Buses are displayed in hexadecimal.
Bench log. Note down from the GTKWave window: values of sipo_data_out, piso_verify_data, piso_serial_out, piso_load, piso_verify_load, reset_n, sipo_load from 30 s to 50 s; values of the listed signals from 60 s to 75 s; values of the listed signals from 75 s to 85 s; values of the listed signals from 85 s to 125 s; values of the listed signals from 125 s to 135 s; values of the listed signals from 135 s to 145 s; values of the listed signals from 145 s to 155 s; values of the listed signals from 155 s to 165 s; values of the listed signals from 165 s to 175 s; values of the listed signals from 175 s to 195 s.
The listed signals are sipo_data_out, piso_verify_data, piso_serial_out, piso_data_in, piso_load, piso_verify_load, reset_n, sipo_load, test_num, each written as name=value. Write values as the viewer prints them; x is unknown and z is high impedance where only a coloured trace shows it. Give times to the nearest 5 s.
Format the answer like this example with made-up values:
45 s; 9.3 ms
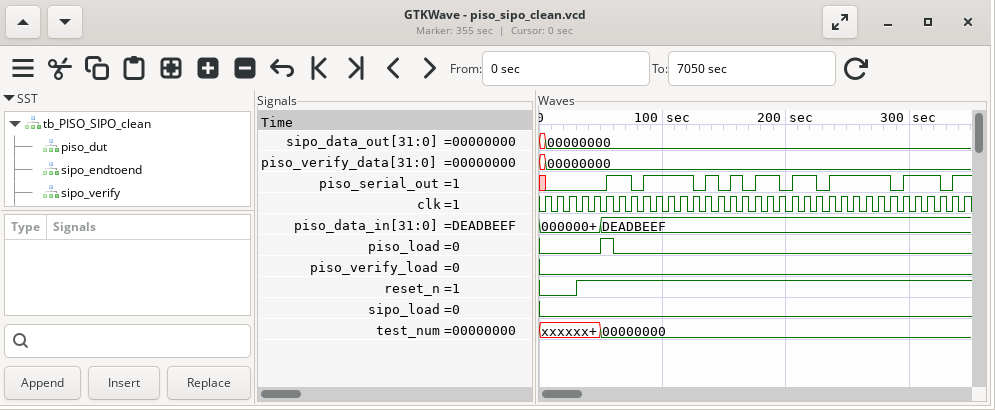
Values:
sipo_data_out=00000000, piso_verify_data=00000000, piso_serial_out=0, piso_load=0, piso_verify_load=0, reset_n=1, sipo_load=0; sipo_data_out=00000000, piso_verify_data=00000000, piso_serial_out=1, piso_data_in=DEADBEEF, piso_load=0, piso_verify_load=0, reset_n=1, sipo_load=0, test_num=00000000; sipo_data_out=00000000, piso_verify_data=00000000, piso_serial_out=0, piso_data_in=DEADBEEF, piso_load=0, piso_verify_load=0, reset_n=1, sipo_load=0, test_num=00000000; sipo_data_out=00000000, piso_verify_data=00000000, piso_serial_out=1, piso_data_in=DEADBEEF, piso_load=0, piso_verify_load=0, reset_n=1, sipo_load=0, test_num=00000000; sipo_data_out=00000000, piso_verify_data=00000000, piso_serial_out=0, piso_data_in=DEADBEEF, piso_load=0, piso_verify_load=0, reset_n=1, sipo_load=0, test_num=00000000; sipo_data_out=00000000, piso_verify_data=00000000, piso_serial_out=1, piso_data_in=DEADBEEF, piso_load=0, piso_verify_load=0, reset_n=1, sipo_load=0, test_num=00000000; sipo_data_out=00000000, piso_verify_data=00000000, piso_serial_out=0, piso_data_in=DEADBEEF, piso_load=0, piso_verify_load=0, reset_n=1, sipo_load=0, test_num=00000000; sipo_data_out=00000000, piso_verify_data=00000000, piso_serial_out=1, piso_data_in=DEADBEEF, piso_load=0, piso_verify_load=0, reset_n=1, sipo_load=0, test_num=00000000; sipo_data_out=00000000, piso_verify_data=00000000, piso_serial_out=0, piso_data_in=DEADBEEF, piso_load=0, piso_verify_load=0, reset_n=1, sipo_load=0, test_num=00000000; sipo_data_out=00000000, piso_verify_data=00000000, piso_serial_out=1, piso_data_in=DEADBEEF, piso_load=0, piso_verify_load=0, reset_n=1, sipo_load=0, test_num=00000000
